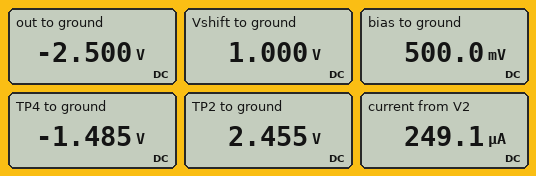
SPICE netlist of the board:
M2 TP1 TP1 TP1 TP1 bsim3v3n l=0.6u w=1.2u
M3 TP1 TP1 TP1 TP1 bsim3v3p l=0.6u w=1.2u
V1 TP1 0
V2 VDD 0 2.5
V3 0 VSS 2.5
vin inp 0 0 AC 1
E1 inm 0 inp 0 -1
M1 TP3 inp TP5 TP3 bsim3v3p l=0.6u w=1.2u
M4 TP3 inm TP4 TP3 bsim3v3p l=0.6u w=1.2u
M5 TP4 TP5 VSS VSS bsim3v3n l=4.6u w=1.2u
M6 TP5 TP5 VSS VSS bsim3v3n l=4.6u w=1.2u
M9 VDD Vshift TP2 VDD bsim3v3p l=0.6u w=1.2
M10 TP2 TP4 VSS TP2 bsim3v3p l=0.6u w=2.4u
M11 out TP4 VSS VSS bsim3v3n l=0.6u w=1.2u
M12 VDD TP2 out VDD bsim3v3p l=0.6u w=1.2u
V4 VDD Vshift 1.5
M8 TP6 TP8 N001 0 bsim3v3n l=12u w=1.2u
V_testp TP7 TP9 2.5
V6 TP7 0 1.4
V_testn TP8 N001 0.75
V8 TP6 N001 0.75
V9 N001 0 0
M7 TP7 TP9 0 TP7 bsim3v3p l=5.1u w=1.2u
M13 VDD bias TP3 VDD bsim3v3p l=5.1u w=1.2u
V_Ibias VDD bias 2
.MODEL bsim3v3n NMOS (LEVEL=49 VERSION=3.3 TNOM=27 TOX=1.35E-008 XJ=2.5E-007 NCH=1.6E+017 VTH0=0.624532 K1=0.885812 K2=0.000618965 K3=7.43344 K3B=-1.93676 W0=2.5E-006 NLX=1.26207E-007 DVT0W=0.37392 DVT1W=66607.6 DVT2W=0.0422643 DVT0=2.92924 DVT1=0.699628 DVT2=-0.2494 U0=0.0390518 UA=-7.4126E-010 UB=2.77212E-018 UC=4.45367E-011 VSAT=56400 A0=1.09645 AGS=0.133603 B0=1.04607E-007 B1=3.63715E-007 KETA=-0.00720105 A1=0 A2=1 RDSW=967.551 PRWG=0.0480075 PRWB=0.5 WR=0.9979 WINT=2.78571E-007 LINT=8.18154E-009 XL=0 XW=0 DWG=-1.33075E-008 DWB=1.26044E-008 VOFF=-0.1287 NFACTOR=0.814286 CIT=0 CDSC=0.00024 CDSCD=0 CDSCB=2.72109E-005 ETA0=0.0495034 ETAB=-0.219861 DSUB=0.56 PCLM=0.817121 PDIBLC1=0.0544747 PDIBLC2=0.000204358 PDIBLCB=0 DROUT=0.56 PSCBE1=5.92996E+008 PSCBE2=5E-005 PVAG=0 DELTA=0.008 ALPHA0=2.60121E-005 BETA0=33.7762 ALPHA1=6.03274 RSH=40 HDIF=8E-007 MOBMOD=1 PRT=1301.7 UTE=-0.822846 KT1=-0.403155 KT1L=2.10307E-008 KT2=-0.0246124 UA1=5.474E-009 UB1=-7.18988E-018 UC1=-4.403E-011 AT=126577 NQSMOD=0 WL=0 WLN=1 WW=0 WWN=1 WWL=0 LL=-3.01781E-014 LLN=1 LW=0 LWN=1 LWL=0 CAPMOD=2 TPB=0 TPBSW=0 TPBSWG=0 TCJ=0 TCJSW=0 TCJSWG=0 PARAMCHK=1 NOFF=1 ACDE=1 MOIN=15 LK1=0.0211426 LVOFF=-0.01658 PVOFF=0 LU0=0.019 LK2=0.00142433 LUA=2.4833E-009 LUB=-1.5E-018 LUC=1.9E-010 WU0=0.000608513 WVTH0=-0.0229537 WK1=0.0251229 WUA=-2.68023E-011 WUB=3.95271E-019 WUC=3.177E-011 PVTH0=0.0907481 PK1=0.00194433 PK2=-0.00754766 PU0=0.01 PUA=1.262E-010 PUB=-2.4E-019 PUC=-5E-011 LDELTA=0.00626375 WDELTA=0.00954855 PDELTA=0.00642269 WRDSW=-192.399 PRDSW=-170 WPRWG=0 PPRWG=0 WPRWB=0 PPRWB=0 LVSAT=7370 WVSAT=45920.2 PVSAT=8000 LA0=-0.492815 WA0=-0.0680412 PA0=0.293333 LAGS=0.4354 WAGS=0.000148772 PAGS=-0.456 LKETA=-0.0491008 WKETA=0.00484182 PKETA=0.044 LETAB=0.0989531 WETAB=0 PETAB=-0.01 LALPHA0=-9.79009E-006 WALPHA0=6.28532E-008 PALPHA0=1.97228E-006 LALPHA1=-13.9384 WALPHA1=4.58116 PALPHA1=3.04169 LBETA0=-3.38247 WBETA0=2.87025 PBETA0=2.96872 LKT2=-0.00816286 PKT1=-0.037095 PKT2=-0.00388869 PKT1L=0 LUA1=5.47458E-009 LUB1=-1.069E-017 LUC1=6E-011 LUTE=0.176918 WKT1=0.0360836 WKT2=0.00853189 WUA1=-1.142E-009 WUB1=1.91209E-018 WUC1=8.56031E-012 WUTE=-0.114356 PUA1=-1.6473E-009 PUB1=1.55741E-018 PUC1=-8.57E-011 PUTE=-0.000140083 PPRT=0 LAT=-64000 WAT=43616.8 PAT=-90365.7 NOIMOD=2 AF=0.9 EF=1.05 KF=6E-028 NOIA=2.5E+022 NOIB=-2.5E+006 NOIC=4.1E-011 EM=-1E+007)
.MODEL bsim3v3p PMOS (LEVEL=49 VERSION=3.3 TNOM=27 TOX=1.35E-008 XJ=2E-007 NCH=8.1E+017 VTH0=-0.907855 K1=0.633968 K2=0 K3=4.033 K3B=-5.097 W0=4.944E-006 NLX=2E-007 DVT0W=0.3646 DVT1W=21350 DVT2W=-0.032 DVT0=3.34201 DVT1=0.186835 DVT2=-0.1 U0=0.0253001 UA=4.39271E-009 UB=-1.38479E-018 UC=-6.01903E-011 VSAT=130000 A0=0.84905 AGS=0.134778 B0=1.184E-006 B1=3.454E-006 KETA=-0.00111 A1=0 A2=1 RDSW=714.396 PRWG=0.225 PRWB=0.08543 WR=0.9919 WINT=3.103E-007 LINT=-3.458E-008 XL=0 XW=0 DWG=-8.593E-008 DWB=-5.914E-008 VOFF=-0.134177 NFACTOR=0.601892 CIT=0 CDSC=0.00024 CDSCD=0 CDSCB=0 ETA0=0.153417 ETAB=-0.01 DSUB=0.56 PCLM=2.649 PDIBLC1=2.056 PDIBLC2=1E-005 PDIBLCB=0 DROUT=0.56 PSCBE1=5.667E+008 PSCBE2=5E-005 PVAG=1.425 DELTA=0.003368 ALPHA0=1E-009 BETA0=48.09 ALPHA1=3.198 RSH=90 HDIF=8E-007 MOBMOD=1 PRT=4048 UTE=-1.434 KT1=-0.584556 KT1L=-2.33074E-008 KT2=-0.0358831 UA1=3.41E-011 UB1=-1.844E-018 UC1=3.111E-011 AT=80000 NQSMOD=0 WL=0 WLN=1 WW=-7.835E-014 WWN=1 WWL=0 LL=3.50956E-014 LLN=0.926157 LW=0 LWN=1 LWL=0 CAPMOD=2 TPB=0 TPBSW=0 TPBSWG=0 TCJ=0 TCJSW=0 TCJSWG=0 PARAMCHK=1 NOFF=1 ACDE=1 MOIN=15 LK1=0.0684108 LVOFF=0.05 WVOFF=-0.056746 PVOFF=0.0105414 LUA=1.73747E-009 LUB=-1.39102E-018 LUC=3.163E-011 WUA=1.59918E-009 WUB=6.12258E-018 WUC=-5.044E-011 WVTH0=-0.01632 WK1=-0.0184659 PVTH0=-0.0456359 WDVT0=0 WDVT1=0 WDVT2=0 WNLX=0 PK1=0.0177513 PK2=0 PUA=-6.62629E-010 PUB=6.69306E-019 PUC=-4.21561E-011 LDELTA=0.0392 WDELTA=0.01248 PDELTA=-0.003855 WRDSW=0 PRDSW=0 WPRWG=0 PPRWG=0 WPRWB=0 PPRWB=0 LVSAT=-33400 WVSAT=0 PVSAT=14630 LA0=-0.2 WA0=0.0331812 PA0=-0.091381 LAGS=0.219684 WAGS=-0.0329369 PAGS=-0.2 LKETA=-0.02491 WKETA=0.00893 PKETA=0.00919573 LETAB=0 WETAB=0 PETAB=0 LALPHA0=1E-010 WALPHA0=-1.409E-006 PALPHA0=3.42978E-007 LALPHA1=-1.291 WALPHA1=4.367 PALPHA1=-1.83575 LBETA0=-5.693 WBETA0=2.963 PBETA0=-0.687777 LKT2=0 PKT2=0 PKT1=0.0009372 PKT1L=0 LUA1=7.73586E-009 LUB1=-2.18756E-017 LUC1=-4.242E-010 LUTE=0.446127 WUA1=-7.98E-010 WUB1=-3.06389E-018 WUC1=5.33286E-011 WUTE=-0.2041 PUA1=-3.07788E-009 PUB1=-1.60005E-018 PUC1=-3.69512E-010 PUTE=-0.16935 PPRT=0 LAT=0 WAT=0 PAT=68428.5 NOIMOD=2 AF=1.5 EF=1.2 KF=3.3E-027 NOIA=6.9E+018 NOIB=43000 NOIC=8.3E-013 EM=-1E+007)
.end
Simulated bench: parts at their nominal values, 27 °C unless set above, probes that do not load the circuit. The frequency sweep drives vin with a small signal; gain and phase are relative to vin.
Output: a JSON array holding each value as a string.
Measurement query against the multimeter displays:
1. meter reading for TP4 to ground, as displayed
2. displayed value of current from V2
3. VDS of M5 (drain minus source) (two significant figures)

["-1.485 V", "249.1 µA", "1.0 V"]
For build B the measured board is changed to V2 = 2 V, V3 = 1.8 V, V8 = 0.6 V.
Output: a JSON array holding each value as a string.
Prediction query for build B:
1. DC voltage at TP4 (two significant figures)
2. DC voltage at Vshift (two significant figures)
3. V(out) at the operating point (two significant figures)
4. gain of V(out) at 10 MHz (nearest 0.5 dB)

["-790 mV", "500 mV", "-1.8 V", "-27.0 dB"]
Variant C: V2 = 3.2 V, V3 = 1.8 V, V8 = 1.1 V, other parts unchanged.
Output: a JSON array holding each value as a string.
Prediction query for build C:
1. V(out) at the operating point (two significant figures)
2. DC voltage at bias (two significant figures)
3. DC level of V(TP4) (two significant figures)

["-1.8 V", "1.2 V", "-780 mV"]
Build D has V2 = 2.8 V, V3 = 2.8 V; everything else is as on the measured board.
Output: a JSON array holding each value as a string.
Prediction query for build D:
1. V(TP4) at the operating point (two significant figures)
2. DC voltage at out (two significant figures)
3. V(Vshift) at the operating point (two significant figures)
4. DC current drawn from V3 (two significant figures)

["-1.8 V", "-2.8 V", "1.3 V", "330 µA"]
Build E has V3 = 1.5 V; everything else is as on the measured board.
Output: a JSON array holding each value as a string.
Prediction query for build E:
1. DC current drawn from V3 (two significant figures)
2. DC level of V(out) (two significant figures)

["130 µA", "-1.5 V"]
